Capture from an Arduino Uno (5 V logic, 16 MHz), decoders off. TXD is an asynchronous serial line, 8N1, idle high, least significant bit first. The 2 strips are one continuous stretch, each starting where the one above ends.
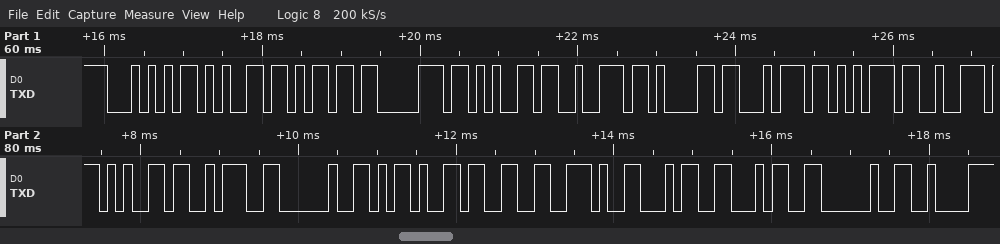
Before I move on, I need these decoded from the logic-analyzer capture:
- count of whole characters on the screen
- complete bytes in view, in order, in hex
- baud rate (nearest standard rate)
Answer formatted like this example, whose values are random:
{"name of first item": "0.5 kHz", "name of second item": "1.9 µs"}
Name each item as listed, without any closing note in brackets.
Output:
{"count of whole characters on the screen": "20", "complete bytes in view, in order, in hex": "0x54 0x65 0x6D 0x70 0x65 0x72 0x61 0x74 0x75 0x72 0x65 0x3A 0x20 0x2D 0x33 0x2E 0x34 0x34 0x20 0xC2", "baud rate": "9600 baud"}
